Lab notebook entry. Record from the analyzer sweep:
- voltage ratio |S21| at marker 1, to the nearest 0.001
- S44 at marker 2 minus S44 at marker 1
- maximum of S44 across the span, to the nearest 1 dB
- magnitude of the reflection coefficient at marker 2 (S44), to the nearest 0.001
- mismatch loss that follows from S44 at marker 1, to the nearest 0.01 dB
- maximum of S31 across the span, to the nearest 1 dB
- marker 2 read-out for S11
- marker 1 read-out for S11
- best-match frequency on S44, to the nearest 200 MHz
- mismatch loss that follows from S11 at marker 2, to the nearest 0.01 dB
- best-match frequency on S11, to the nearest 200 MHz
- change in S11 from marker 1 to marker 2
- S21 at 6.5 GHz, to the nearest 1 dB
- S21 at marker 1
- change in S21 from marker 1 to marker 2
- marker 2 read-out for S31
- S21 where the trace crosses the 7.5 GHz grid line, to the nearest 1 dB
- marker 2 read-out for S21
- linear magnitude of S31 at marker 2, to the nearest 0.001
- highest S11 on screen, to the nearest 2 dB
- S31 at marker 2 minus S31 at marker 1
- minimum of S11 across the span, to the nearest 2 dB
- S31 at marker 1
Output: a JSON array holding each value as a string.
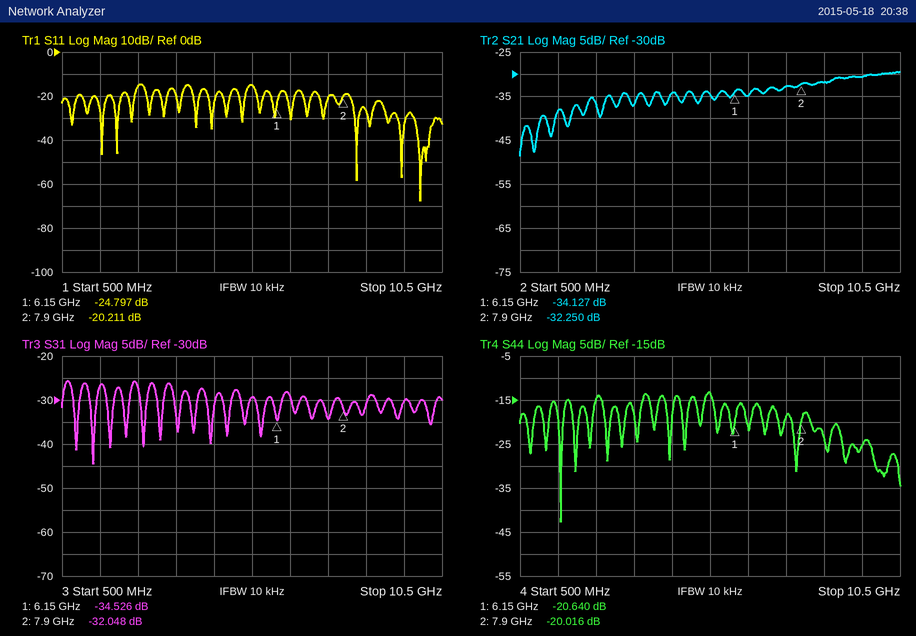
["0.020", "0.624 dB", "-13 dB", "0.100", "0.04 dB", "-26 dB", "-20.211 dB", "-24.797 dB", "1.6 GHz", "0.04 dB", "10.0 GHz", "4.586 dB", "-35 dB", "-34.127 dB", "1.877 dB", "-32.048 dB", "-33 dB", "-32.250 dB", "0.025", "-14 dB", "2.478 dB", "-68 dB", "-34.526 dB"]
